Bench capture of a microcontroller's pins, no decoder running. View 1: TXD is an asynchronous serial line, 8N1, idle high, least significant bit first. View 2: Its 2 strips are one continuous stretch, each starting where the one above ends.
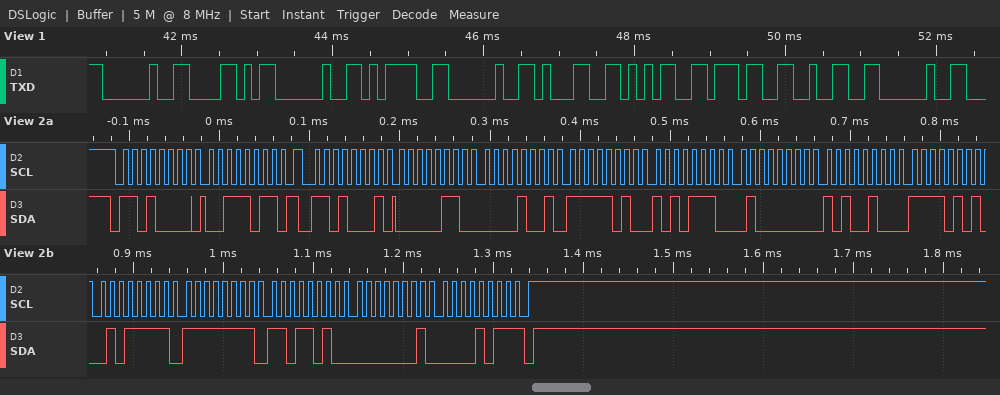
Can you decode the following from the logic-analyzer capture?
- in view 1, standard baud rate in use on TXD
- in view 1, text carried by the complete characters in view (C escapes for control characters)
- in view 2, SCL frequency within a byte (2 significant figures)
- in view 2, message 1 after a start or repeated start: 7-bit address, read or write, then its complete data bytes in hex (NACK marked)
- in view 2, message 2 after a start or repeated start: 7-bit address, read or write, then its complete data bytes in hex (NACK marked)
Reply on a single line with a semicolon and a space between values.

9600 baud; " X = 1572 "; 100 kHz; 0x68 write: 3B; 0x68 read: 06 09 FA AE 40 A4 F5 5F FF DA 01 0B NACK
